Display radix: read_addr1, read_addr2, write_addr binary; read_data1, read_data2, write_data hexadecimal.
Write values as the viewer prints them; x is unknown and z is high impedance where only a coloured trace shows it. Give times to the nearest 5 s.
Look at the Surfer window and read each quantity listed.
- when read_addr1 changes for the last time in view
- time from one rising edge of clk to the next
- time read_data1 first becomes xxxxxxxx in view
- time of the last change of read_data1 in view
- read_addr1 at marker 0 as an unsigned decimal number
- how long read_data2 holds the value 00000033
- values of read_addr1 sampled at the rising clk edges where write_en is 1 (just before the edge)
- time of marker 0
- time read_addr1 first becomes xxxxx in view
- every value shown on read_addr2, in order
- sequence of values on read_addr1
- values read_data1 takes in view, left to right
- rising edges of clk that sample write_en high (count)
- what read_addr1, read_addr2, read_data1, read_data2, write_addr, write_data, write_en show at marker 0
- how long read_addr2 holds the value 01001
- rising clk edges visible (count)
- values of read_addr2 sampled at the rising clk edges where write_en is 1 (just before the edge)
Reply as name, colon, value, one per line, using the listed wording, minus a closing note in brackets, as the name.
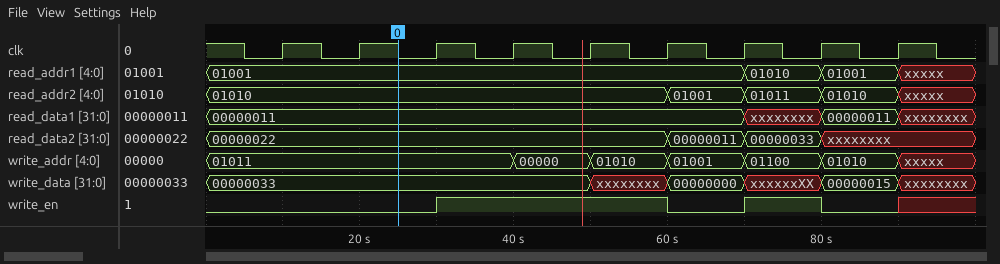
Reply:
when read_addr1 changes for the last time in view: 90 s
time from one rising edge of clk to the next: 10 s
time read_data1 first becomes xxxxxxxx in view: 70 s
time of the last change of read_data1 in view: 90 s
read_addr1 at marker 0 as an unsigned decimal number: 9
how long read_data2 holds the value 00000033: 10 s
values of read_addr1 sampled at the rising clk edges where write_en is 1: 01001, 01001, 01001, 01010
time of marker 0: 25 s
time read_addr1 first becomes xxxxx in view: 90 s
every value shown on read_addr2, in order: 01010, 01001, 01011, 01010, xxxxx
sequence of values on read_addr1: 01001, 01010, 01001, xxxxx
values read_data1 takes in view, left to right: 00000011, xxxxxxxx, 00000011, xxxxxxxx
rising edges of clk that sample write_en high: 4
what read_addr1, read_addr2, read_data1, read_data2, write_addr, write_data, write_en show at marker 0: read_addr1=01001, read_addr2=01010, read_data1=00000011, read_data2=00000022, write_addr=01011, write_data=00000033, write_en=0
how long read_addr2 holds the value 01001: 10 s
rising clk edges visible: 9
values of read_addr2 sampled at the rising clk edges where write_en is 1: 01010, 01010, 01010, 01011
